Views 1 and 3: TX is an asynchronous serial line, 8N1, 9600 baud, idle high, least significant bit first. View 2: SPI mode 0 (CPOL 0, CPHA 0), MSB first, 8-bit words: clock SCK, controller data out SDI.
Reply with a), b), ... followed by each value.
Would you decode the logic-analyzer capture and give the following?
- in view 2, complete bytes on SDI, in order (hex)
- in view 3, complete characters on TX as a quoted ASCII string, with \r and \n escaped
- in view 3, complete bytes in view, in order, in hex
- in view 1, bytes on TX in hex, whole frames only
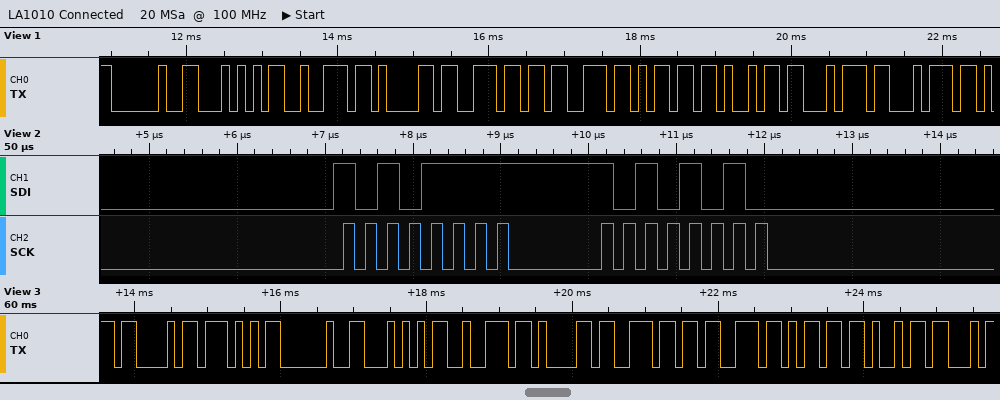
a) 0xAF 0xAA
b) "CW Transmi"
c) 43 57 20 54 72 61 6E 73 6D 69
d) 0x20 0x54 0x72 0x61 0x6E 0x73 0x6D 0x69 0x74 0x74
